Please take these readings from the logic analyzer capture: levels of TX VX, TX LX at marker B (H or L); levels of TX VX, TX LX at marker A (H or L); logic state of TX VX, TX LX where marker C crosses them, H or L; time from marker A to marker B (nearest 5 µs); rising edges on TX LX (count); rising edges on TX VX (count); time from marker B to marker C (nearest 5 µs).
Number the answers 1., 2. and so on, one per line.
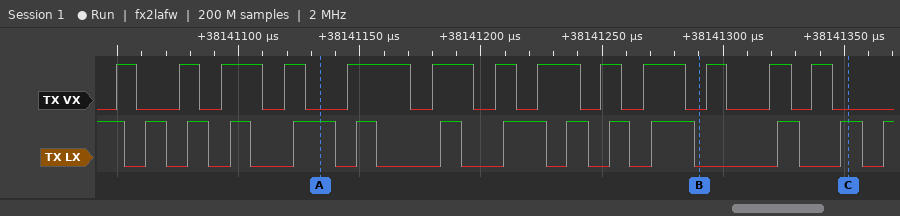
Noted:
1. TX VX=L, TX LX=L
2. TX VX=L, TX LX=H
3. TX VX=L, TX LX=H
4. 155 µs
5. 13
6. 13
7. 60 µs
